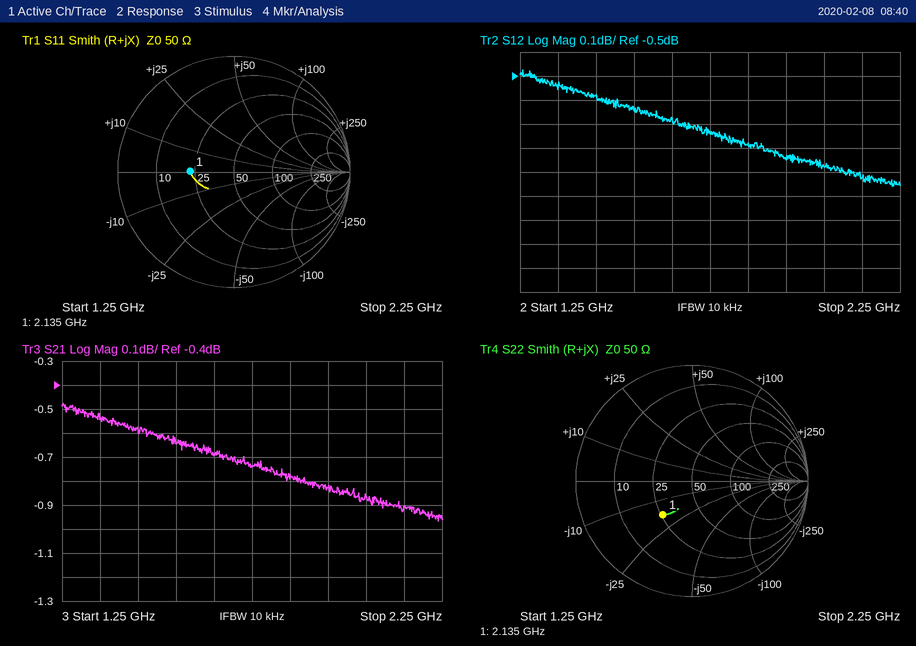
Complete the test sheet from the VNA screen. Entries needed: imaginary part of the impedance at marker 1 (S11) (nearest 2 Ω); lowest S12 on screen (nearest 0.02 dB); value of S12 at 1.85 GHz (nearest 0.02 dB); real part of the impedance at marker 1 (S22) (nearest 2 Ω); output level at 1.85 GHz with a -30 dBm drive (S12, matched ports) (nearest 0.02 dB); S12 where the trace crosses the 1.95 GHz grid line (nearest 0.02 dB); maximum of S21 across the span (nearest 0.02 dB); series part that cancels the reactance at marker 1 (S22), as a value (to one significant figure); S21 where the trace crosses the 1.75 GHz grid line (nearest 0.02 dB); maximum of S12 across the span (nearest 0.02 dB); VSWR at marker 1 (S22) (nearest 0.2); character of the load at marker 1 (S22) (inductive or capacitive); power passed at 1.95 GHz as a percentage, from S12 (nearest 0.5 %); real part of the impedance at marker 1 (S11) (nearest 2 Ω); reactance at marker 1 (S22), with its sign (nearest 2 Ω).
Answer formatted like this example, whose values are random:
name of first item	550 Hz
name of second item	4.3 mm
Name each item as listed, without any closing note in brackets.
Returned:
imaginary part of the impedance at marker 1 (S11)	0 Ω
lowest S12 on screen	-0.96 dB
value of S12 at 1.85 GHz	-0.78 dB
real part of the impedance at marker 1 (S22)	26 Ω
output level at 1.85 GHz with a -30 dBm drive (S12, matched ports)	-30.78 dBm
S12 where the trace crosses the 1.95 GHz grid line	-0.84 dB
maximum of S21 across the span	-0.48 dB
series part that cancels the reactance at marker 1 (S22), as a value	1 nH
S21 where the trace crosses the 1.75 GHz grid line	-0.74 dB
maximum of S12 across the span	-0.48 dB
VSWR at marker 1 (S22)	2.2
character of the load at marker 1 (S22)	capacitive
power passed at 1.95 GHz as a percentage, from S12	82.5 %
real part of the impedance at marker 1 (S11)	22 Ω
reactance at marker 1 (S22), with its sign	-18 Ω
